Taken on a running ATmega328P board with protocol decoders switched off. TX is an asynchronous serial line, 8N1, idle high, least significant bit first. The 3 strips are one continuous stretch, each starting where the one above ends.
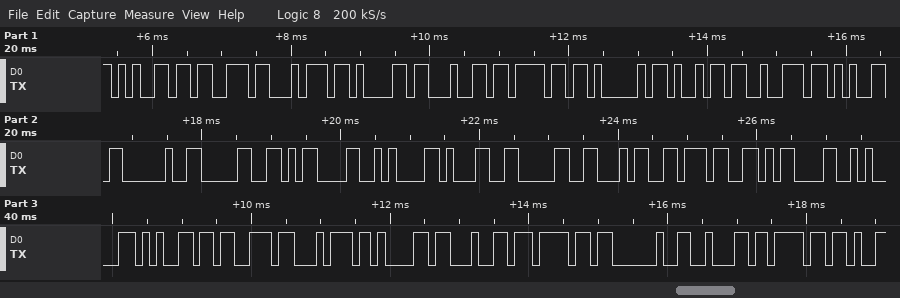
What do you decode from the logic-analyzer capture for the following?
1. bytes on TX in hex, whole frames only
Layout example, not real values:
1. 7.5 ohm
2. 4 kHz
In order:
1. 0x65 0x73 0x74 0x61 0x64 0x6F 0x41 0x69 0x72 0x65 0x20 0x30 0x0D 0x0A 0x31 0x30 0x34 0x37 0x0D 0x0A 0x65 0x73 0x74 0x61 0x64 0x6F 0x20 0x62 0x6F
